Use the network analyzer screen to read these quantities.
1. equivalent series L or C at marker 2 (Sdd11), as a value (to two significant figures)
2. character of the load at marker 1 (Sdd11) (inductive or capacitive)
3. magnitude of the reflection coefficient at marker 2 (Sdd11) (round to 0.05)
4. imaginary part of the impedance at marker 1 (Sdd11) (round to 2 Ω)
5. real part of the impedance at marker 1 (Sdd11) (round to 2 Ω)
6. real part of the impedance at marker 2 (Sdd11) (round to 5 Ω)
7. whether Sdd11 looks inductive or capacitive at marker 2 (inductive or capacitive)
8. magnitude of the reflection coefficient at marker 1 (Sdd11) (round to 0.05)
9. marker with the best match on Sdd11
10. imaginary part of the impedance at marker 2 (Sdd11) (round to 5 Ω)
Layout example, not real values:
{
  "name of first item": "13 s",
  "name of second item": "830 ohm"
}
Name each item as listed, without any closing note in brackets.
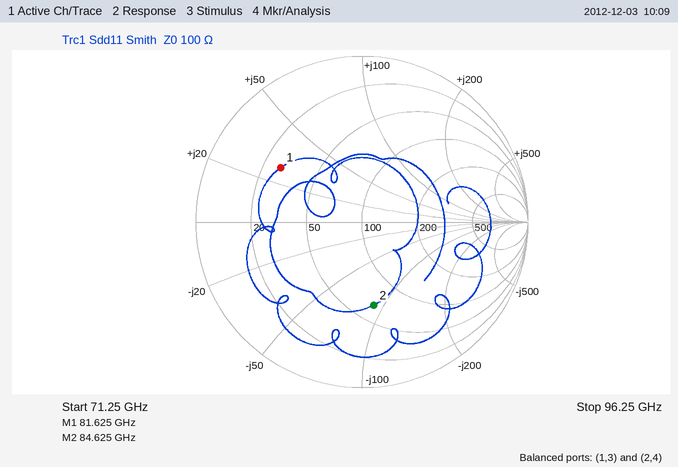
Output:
{
  "equivalent series L or C at marker 2 (Sdd11), as a value": "21 fF",
  "character of the load at marker 1 (Sdd11)": "inductive",
  "magnitude of the reflection coefficient at marker 2 (Sdd11)": "0.50",
  "imaginary part of the impedance at marker 1 (Sdd11)": "+28 Ω",
  "real part of the impedance at marker 1 (Sdd11)": "28 Ω",
  "real part of the impedance at marker 2 (Sdd11)": "65 Ω",
  "whether Sdd11 looks inductive or capacitive at marker 2": "capacitive",
  "magnitude of the reflection coefficient at marker 1 (Sdd11)": "0.60",
  "marker with the best match on Sdd11": "marker 2",
  "imaginary part of the impedance at marker 2 (Sdd11)": "-90 Ω"
}
